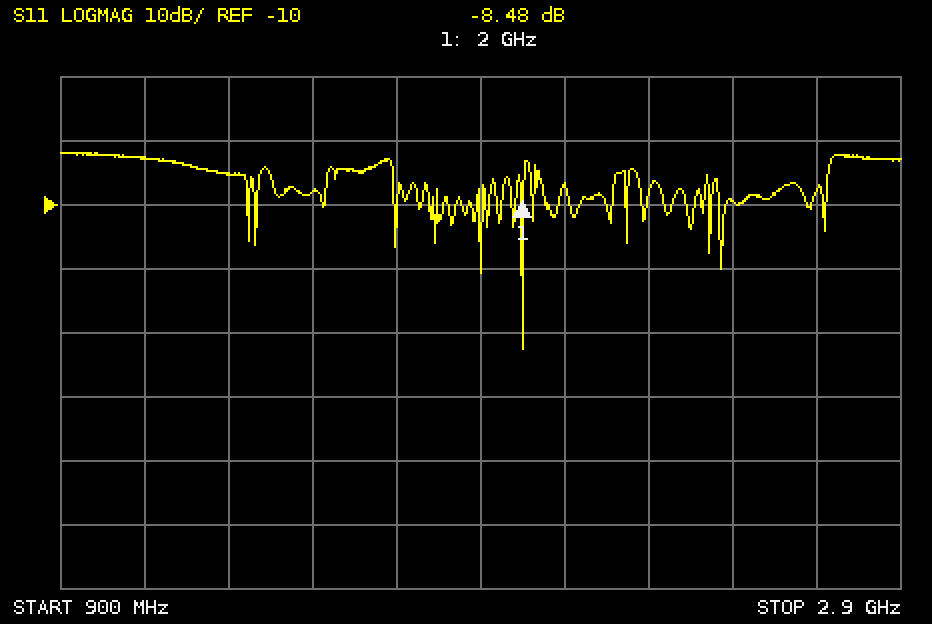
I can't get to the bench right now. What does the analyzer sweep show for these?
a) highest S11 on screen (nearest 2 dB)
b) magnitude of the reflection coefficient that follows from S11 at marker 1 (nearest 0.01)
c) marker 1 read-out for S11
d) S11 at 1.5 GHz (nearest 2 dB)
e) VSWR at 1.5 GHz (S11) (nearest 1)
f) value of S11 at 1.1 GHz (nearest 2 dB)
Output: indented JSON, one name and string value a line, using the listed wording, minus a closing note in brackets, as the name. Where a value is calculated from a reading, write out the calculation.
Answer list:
{
  "highest S11 on screen": "-2 dB",
  "magnitude of the reflection coefficient that follows from S11 at marker 1": "10^(-8.48/20) ≈ 0.38",
  "marker 1 read-out for S11": "-8.48 dB",
  "S11 at 1.5 GHz": "-8 dB",
  "VSWR at 1.5 GHz (S11)": "|Γ| = 10^(-8/20) = 0.3981; VSWR = (1 + 0.3981)/(1 − 0.3981) ≈ 2",
  "value of S11 at 1.1 GHz": "-2 dB"
}
